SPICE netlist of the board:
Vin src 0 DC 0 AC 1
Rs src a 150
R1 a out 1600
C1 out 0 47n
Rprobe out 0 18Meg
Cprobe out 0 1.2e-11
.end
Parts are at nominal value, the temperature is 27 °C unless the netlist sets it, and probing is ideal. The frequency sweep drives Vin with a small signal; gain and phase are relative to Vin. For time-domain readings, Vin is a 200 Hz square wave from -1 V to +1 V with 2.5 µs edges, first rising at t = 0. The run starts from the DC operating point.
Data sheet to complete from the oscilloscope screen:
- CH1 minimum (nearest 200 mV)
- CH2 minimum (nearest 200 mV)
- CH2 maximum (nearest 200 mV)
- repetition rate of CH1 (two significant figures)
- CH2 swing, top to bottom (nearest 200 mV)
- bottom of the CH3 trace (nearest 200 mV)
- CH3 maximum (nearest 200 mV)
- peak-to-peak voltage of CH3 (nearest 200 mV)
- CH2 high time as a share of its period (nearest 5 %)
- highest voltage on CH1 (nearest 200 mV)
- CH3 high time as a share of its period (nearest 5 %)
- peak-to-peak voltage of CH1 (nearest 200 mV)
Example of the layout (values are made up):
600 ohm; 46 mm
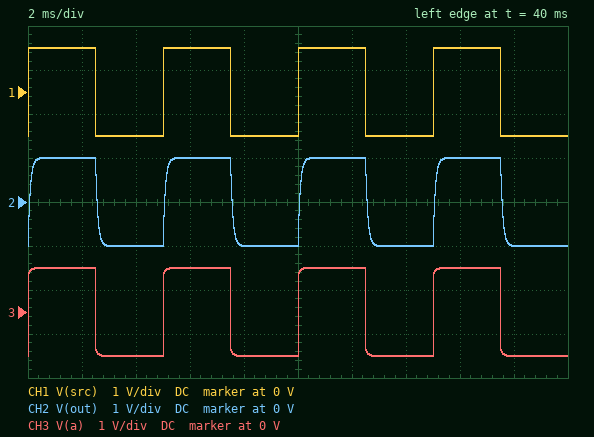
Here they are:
-1.0 V; -1.0 V; 1.0 V; 200 Hz; 2.0 V; -1.0 V; 1.0 V; 2.0 V; 50 %; 1.0 V; 50 %; 2.0 V
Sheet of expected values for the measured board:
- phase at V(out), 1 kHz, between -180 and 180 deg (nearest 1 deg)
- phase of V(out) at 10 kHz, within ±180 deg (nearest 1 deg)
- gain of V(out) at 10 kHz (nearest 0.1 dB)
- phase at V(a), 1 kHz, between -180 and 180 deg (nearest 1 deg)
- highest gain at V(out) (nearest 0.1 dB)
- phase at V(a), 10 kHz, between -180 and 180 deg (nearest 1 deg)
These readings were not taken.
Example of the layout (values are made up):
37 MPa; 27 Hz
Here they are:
-27 deg; -79 deg; -14.4 dB; -2 deg; 0 dB; -1 deg
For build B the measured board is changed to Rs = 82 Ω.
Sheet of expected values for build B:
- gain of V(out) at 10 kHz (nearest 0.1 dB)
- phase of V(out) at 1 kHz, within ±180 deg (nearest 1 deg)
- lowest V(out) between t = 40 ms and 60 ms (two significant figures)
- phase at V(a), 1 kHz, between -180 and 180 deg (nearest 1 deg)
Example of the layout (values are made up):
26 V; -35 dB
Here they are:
-14.1 dB; -26 deg; -1.0 V; -1 deg
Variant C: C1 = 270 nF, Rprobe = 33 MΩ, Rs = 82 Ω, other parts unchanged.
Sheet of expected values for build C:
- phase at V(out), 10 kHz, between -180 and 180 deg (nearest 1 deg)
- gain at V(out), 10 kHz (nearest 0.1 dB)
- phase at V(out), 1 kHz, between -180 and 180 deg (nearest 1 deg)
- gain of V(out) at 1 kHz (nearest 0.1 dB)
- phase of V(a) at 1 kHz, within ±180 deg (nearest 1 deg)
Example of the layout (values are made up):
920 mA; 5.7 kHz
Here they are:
-88 deg; -29.1 dB; -71 deg; -9.6 dB; -1 deg
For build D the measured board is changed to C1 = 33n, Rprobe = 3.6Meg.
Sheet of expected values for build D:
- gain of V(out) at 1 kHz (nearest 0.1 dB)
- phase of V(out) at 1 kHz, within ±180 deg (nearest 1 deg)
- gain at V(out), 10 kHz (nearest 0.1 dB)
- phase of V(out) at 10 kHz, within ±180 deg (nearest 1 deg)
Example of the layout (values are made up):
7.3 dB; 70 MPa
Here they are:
-0.5 dB; -20 deg; -11.5 dB; -75 deg
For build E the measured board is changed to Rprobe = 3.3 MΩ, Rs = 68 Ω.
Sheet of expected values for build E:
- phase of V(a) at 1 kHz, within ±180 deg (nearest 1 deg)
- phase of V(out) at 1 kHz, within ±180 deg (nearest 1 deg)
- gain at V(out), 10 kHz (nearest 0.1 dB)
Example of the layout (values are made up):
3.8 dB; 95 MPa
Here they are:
-1 deg; -26 deg; -14.0 dB
